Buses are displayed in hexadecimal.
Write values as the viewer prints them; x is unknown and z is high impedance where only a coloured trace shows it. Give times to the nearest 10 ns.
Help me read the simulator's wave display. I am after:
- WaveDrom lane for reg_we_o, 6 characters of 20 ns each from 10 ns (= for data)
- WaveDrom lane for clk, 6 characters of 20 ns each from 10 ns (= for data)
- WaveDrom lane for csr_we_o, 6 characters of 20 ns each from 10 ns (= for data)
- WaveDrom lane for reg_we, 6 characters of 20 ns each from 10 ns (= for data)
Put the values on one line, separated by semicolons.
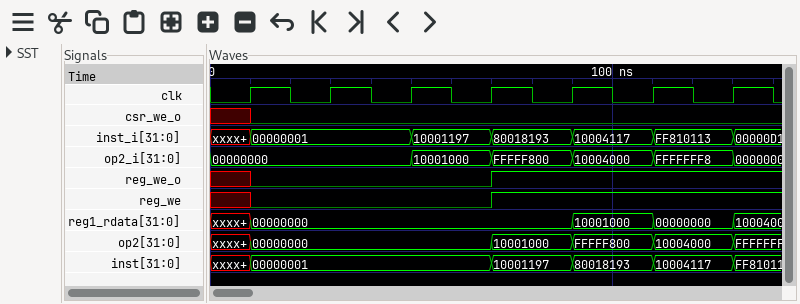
{name: 'reg_we_o', wave: '0..1..'}; {name: 'clk', wave: 'p.....'}; {name: 'csr_we_o', wave: '0.....'}; {name: 'reg_we', wave: '0..1..'}
